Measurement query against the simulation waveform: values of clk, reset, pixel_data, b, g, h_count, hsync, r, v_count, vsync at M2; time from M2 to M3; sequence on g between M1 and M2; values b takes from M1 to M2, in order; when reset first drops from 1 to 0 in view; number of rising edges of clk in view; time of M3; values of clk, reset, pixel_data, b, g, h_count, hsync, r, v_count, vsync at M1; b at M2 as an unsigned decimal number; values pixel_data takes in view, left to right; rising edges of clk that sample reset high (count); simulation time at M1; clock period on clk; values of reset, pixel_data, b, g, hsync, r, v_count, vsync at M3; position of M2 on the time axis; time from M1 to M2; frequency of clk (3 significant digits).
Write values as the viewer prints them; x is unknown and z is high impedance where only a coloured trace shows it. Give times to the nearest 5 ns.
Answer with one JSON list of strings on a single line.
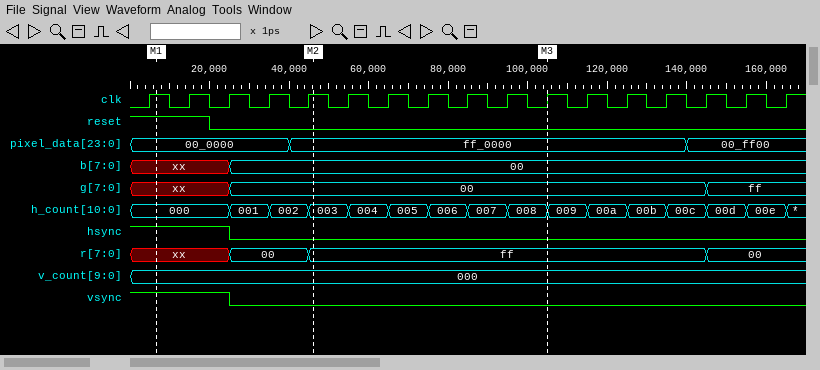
["clk=1, reset=0, pixel_data=ff_0000, b=00, g=00, h_count=003, hsync=0, r=ff, v_count=000, vsync=0", "60 ns", "xx, 00", "xx, 00", "20 ns", "17", "105 ns", "clk=1, reset=1, pixel_data=00_0000, b=xx, g=xx, h_count=000, hsync=1, r=xx, v_count=000, vsync=1", "0", "00_0000, ff_0000, 00_ff00", "2", "5 ns", "10 ns", "reset=0, pixel_data=ff_0000, b=00, g=00, hsync=0, r=ff, v_count=000, vsync=0", "45 ns", "40 ns", "100 MHz"]
